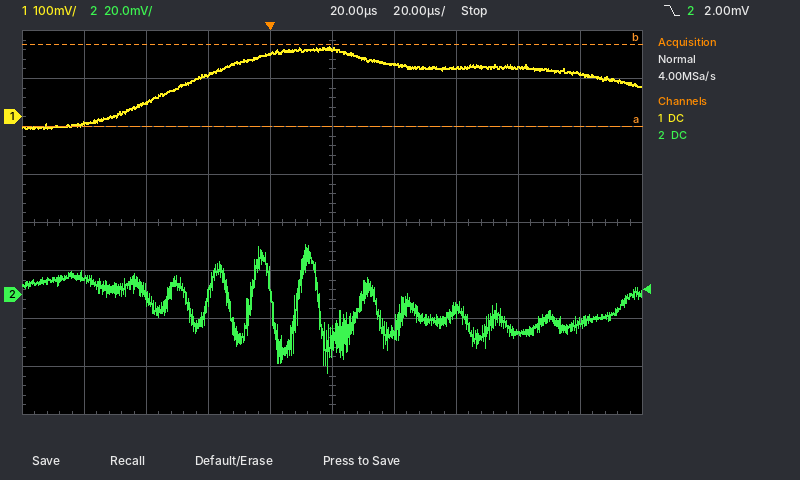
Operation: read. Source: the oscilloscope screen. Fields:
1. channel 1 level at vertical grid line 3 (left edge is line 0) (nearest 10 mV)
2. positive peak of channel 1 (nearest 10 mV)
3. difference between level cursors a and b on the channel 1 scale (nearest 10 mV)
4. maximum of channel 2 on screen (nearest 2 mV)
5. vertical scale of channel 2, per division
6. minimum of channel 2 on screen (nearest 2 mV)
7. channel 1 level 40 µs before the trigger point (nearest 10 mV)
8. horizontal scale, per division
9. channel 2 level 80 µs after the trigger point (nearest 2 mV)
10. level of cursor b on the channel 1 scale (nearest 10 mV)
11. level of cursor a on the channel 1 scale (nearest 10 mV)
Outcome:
90 mV
150 mV
170 mV
20 mV
20 mV
-32 mV
30 mV
20 µs
-16 mV
150 mV
-20 mV
